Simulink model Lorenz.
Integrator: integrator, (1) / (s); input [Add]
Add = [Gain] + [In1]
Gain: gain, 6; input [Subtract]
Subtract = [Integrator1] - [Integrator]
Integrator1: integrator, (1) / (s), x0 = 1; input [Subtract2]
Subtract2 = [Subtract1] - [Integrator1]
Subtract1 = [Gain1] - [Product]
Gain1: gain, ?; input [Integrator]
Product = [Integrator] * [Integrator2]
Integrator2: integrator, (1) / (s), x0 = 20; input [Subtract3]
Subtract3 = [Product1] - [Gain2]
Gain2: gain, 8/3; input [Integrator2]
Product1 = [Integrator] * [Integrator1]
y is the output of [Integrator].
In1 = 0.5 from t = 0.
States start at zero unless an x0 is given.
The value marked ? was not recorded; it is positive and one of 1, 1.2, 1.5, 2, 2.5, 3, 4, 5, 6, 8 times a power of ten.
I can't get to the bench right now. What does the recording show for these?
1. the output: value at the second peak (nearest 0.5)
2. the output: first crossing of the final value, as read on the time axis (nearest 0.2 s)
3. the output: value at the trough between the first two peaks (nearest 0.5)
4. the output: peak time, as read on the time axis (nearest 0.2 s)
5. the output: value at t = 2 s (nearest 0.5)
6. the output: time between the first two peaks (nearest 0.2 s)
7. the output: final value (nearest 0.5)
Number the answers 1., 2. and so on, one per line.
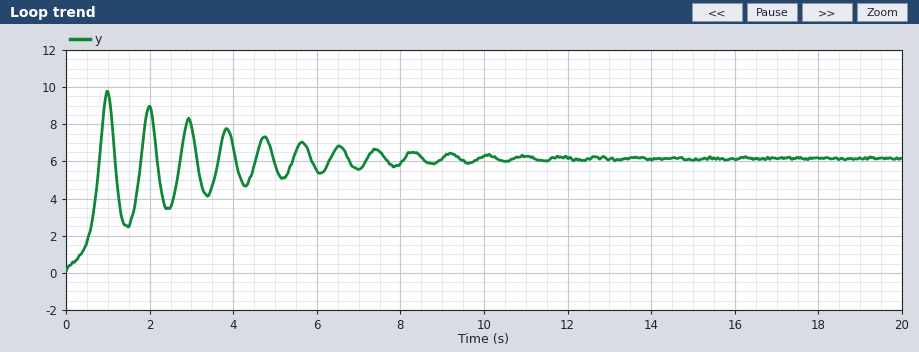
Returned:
1. 9.0
2. 0.8 s
3. 2.5
4. 1.0 s
5. 9.0
6. 1.0 s
7. 6.0
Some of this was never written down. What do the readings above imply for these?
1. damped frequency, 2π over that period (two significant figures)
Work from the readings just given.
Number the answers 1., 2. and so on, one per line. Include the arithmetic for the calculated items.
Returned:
1. 2π / 1 = 6.3 rad/s
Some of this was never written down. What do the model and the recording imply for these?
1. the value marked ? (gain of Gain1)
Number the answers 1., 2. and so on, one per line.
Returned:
1. 15
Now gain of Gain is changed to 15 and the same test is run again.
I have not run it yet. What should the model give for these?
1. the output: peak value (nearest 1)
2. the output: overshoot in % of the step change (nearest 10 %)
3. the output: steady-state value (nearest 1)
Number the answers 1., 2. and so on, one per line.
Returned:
1. 11
2. 70 %
3. 6
